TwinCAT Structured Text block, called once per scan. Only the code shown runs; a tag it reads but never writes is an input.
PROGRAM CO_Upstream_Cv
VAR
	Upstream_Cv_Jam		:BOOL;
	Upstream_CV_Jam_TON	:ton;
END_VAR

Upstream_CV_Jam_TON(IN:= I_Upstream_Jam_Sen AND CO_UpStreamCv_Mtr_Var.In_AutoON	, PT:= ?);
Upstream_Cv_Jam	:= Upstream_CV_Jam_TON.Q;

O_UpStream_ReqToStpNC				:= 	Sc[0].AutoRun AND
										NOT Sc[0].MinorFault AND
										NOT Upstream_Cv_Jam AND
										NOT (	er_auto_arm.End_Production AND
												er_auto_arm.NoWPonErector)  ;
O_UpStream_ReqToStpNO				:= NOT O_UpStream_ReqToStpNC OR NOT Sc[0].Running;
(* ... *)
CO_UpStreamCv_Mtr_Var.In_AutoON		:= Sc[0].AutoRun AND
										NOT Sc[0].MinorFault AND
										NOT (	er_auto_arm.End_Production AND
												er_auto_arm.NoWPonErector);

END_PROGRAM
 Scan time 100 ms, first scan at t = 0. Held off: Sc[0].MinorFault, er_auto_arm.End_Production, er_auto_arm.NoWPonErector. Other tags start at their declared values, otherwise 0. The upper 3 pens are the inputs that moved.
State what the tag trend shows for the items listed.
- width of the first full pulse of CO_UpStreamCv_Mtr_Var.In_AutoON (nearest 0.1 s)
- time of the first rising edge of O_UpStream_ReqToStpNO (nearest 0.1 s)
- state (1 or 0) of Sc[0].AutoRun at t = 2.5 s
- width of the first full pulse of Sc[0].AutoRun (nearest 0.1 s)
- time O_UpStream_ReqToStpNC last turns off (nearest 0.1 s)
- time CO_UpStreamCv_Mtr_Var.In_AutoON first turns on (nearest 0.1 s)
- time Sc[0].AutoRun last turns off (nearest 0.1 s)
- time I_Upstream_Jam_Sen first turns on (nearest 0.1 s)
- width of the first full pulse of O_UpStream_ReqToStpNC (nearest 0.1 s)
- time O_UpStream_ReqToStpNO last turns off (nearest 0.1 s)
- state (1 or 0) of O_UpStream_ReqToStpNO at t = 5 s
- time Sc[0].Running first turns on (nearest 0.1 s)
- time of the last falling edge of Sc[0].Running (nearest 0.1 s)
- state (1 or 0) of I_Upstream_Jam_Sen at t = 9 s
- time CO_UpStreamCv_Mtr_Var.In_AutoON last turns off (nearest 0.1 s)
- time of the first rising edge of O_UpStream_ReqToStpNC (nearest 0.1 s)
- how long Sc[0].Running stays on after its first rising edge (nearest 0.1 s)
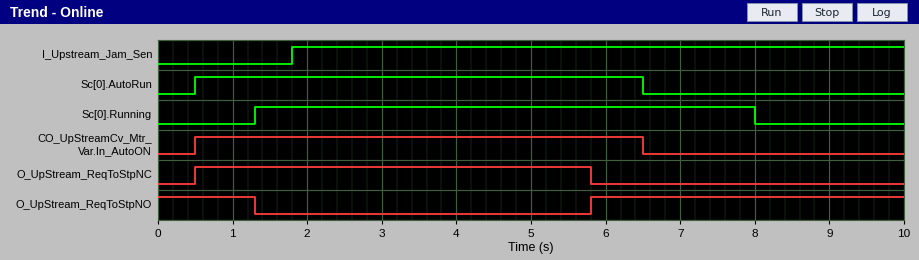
6.0 s
5.8 s
1
6.0 s
5.8 s
0.5 s
6.5 s
1.8 s
5.3 s
1.3 s
0
1.3 s
8.0 s
1
6.5 s
0.5 s
6.7 s
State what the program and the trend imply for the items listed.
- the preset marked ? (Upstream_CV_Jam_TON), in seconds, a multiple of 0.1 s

4.0 s
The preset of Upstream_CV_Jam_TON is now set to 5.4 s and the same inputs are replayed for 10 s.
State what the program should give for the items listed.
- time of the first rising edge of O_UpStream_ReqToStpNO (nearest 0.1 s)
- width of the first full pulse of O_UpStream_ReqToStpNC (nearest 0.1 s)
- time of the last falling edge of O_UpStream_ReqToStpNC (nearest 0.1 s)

6.5 s
6.0 s
6.5 s
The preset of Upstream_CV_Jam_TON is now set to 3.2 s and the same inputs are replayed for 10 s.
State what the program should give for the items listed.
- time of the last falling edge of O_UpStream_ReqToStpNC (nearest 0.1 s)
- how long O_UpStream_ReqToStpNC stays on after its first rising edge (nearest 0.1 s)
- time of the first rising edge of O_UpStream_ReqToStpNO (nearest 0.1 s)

5.0 s
4.5 s
5.0 s
